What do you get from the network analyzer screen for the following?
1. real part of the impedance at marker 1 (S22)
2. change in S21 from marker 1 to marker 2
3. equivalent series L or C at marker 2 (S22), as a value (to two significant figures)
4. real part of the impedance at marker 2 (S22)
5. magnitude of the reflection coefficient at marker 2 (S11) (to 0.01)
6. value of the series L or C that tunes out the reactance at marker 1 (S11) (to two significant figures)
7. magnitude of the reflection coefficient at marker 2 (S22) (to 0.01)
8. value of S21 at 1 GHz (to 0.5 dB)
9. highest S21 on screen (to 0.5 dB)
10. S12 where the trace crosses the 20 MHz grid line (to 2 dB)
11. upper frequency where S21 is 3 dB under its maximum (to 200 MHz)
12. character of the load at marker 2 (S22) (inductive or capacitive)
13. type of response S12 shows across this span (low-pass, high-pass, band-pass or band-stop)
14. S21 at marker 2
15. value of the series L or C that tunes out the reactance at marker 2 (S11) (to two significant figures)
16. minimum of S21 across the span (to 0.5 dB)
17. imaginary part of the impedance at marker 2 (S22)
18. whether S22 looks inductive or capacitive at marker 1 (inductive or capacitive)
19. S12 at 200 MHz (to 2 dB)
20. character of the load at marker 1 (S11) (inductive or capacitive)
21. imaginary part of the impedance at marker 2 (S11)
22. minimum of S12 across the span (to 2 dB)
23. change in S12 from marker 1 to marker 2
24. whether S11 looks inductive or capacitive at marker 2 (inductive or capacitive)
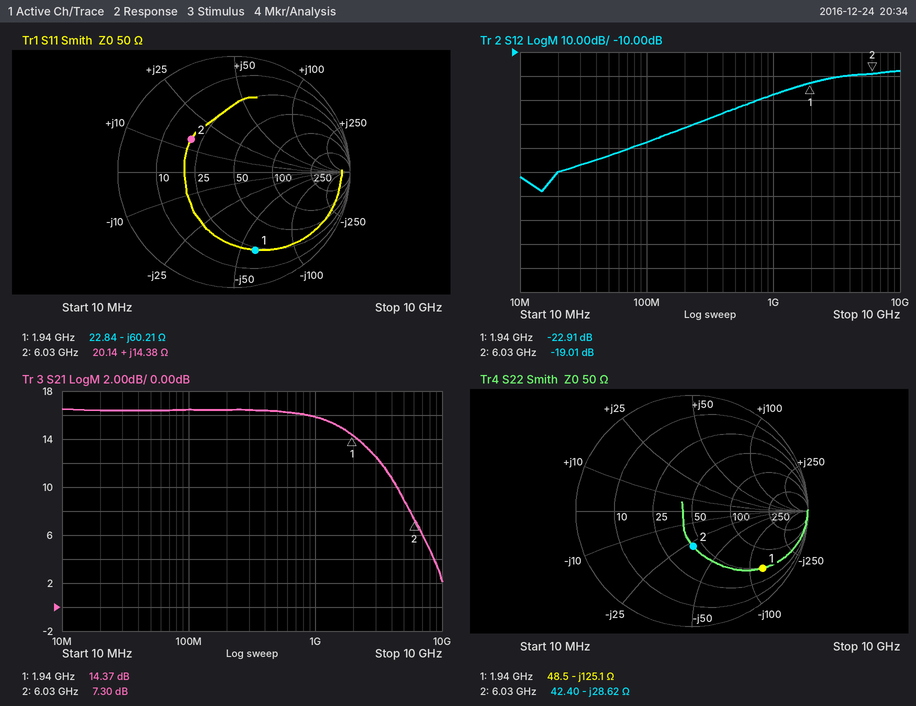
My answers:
48.5 Ω
-7.07 dB
920 fF
42.40 Ω
0.46
4.9 nH
0.31
16.0 dB
16.5 dB
-60 dB
2.4 GHz
capacitive
high-pass
7.30 dB
1.8 pF
2.0 dB
-28.62 Ω
capacitive
-42 dB
capacitive
+14.38 Ω
-68 dB
3.90 dB
inductive
